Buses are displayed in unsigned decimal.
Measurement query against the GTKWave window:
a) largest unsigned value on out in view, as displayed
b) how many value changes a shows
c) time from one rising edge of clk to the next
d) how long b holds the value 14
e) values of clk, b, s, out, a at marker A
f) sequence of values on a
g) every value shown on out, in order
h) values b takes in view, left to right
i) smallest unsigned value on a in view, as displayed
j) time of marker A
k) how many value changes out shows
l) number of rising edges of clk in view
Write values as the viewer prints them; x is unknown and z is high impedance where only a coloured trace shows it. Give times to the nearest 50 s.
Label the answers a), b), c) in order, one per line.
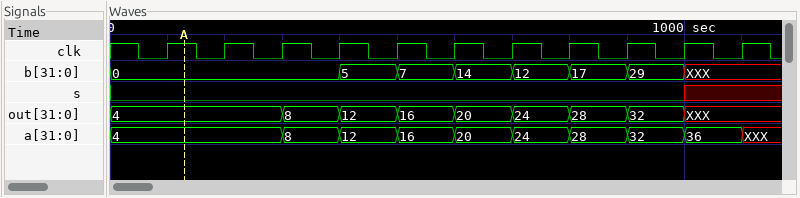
a) 32
b) 9
c) 100 s
d) 100 s
e) clk=1, b=0, s=0, out=4, a=4
f) 4, 8, 12, 16, 20, 24, 28, 32, 36, XXX
g) 4, 8, 12, 16, 20, 24, 28, 32, XXX
h) 0, 5, 7, 14, 12, 17, 29, XXX
i) 4
j) 150 s
k) 8
l) 11
